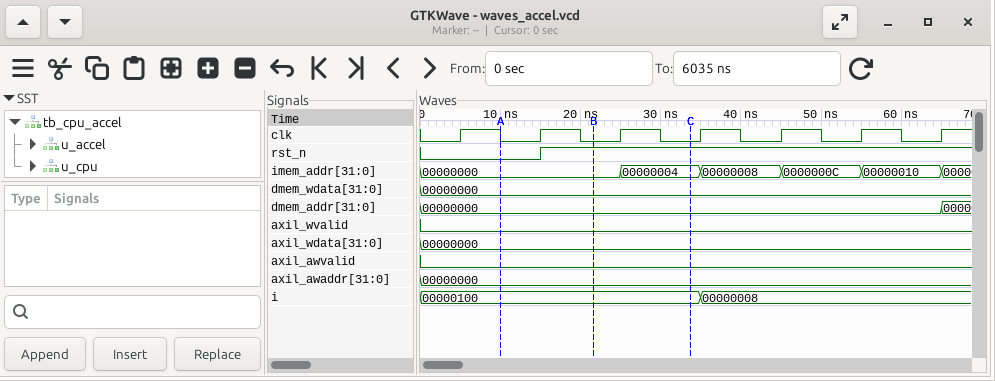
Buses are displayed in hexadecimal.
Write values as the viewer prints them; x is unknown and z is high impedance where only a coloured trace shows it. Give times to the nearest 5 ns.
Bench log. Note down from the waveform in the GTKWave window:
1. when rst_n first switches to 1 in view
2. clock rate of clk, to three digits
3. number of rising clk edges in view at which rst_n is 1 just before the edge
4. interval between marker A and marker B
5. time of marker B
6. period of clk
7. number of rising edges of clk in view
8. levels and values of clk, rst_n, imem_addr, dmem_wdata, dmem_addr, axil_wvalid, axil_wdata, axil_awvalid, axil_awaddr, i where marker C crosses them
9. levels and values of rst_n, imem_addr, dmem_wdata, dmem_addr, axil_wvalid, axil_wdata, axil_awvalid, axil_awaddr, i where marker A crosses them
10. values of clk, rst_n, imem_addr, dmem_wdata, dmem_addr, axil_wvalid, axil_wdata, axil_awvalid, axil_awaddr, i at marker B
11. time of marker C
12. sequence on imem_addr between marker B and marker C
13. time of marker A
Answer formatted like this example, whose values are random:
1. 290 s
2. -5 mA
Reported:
1. 15 ns
2. 100 MHz
3. 5
4. 10 ns
5. 20 ns
6. 10 ns
7. 7
8. clk=0, rst_n=1, imem_addr=00000004, dmem_wdata=00000000, dmem_addr=00000000, axil_wvalid=0, axil_wdata=00000000, axil_awvalid=0, axil_awaddr=00000000, i=00000100
9. rst_n=0, imem_addr=00000000, dmem_wdata=00000000, dmem_addr=00000000, axil_wvalid=0, axil_wdata=00000000, axil_awvalid=0, axil_awaddr=00000000, i=00000100
10. clk=0, rst_n=1, imem_addr=00000000, dmem_wdata=00000000, dmem_addr=00000000, axil_wvalid=0, axil_wdata=00000000, axil_awvalid=0, axil_awaddr=00000000, i=00000100
11. 35 ns
12. 00000000, 00000004
13. 10 ns
